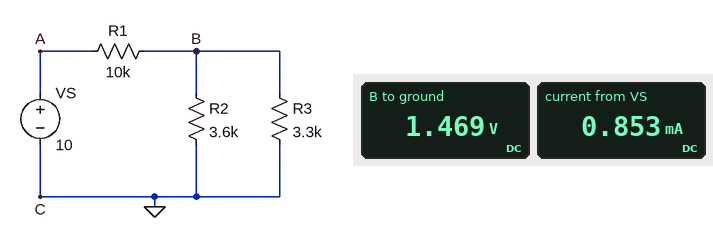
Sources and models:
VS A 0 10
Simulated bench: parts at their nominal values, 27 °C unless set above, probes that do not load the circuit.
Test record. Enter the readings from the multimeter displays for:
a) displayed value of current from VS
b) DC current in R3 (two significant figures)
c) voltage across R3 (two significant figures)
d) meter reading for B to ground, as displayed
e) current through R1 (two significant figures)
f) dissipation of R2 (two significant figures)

0.853 mA
450 µA
1.5 V
1.469 V
850 µA
600 µW
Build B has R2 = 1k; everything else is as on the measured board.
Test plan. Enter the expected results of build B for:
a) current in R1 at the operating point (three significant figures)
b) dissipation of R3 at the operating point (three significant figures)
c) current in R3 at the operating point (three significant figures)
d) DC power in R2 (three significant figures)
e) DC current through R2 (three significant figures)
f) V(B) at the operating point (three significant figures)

929 µA
154 µW
216 µA
508 µW
713 µA
713 mV
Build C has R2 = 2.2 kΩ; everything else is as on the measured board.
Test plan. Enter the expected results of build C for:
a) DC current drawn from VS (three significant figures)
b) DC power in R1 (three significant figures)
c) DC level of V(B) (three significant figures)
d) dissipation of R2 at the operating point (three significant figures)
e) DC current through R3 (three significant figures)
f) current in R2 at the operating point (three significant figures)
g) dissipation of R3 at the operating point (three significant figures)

883 µA
7.80 mW
1.17 V
618 µW
353 µA
530 µA
412 µW
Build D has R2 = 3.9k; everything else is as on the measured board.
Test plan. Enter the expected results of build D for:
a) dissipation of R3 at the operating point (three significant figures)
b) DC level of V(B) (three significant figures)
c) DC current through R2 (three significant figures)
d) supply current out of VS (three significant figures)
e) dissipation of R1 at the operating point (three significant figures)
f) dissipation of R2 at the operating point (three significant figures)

697 µW
1.52 V
389 µA
848 µA
7.20 mW
590 µW
